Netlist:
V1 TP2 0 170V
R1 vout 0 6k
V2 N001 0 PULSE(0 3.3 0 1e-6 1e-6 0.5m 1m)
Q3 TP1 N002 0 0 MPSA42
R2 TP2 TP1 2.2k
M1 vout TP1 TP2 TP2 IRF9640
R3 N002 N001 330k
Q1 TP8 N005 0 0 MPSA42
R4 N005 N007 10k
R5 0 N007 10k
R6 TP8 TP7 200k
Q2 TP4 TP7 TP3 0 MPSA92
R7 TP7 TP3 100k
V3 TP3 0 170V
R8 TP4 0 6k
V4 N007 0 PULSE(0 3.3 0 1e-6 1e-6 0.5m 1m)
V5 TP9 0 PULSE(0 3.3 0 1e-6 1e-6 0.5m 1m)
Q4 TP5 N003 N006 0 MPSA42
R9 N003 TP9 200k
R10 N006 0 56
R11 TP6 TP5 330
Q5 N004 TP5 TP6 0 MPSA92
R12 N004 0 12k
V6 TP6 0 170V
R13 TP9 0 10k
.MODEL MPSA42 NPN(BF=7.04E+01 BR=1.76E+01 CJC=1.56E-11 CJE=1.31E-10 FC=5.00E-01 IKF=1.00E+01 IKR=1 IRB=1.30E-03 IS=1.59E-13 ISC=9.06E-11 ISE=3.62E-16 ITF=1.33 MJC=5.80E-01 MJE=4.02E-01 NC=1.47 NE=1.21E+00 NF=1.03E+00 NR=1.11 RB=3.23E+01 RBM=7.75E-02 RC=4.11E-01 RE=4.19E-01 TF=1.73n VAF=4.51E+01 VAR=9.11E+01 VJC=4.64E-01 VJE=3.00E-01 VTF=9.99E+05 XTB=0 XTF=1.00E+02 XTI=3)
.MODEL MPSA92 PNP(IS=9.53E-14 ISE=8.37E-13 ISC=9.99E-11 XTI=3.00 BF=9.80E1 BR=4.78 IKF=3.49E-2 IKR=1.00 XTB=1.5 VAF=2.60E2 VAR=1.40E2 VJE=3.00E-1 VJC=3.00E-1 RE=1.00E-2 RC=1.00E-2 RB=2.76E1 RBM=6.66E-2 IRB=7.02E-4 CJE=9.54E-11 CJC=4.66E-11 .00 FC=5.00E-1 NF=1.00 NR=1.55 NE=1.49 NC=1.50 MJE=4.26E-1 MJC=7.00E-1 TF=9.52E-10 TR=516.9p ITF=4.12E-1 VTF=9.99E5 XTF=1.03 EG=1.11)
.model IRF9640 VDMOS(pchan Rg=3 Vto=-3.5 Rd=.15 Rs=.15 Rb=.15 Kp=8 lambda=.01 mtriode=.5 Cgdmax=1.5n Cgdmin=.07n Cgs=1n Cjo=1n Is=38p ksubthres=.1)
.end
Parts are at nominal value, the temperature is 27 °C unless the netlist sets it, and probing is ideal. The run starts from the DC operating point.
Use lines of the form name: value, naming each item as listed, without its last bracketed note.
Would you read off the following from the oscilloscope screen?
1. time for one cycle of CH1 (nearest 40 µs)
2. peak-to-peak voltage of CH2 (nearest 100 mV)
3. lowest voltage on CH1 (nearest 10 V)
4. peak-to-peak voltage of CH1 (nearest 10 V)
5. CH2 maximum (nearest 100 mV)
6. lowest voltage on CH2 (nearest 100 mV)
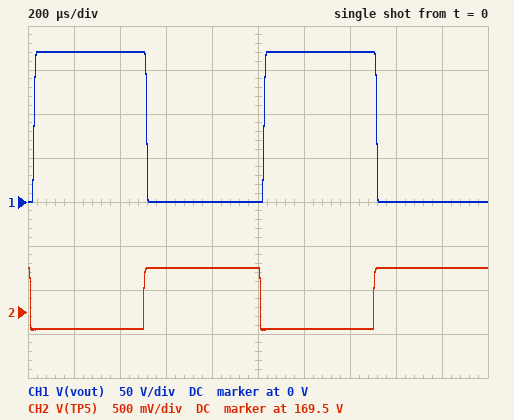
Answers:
time for one cycle of CH1: 1.00 ms
peak-to-peak voltage of CH2: 700 mV
lowest voltage on CH1: 0 V
peak-to-peak voltage of CH1: 170 V
CH2 maximum: 170.0 V
lowest voltage on CH2: 169.3 V
